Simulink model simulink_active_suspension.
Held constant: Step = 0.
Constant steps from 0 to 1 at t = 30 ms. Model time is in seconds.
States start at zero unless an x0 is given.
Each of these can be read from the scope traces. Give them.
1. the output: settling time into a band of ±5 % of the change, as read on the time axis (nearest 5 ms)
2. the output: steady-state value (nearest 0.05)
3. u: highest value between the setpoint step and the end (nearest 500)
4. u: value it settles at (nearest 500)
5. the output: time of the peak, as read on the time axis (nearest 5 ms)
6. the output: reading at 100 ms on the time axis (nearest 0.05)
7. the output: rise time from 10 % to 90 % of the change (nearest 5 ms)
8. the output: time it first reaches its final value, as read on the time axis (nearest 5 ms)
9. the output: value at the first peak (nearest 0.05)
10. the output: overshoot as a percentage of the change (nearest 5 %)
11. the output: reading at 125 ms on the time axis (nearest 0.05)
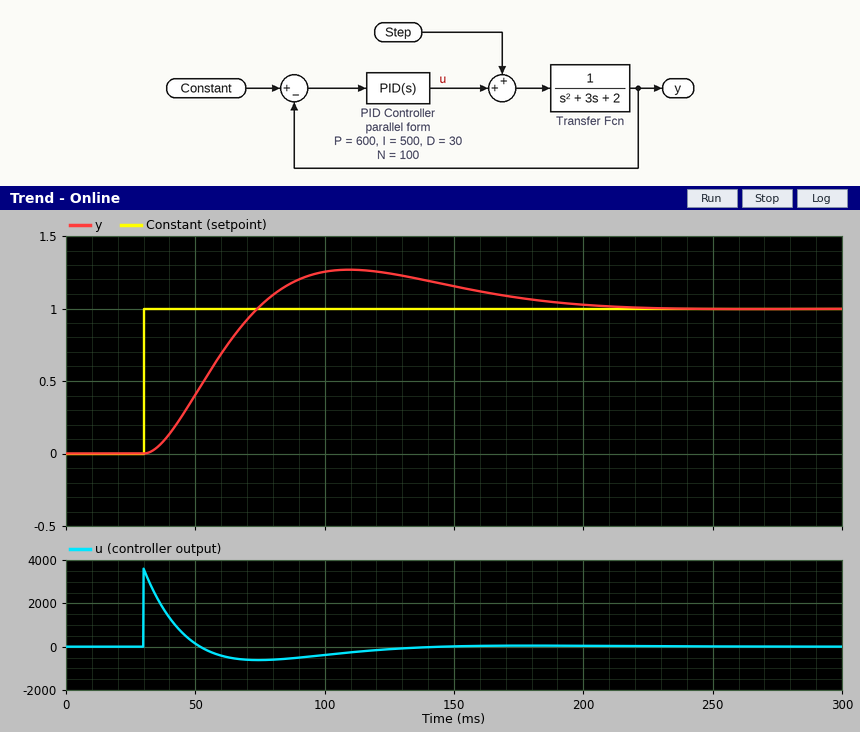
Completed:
185 ms
1.00
3500
0
110 ms
1.25
30 ms
75 ms
1.25
25 %
1.25
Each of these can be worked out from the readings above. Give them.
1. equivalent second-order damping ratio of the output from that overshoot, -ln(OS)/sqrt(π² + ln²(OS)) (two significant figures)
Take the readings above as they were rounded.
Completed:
0.40
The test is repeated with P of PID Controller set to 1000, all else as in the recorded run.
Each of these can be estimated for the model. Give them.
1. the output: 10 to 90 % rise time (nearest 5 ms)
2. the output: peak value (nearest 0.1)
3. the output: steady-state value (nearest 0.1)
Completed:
25 ms
1.4
1.0
